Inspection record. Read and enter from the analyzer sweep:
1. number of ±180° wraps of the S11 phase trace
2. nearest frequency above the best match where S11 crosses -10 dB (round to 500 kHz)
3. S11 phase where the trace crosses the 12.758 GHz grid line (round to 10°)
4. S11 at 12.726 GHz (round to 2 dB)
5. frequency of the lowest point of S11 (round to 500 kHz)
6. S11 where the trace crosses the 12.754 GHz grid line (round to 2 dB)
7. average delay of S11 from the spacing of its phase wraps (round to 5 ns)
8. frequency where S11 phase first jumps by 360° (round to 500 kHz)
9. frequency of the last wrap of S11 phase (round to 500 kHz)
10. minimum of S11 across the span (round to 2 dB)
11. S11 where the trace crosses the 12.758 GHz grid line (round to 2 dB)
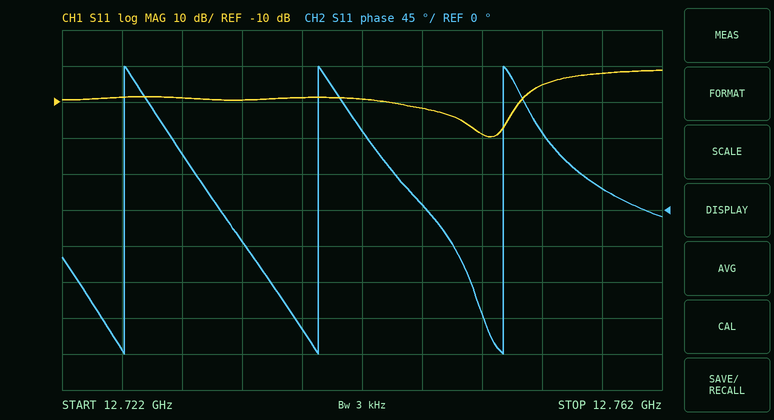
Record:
3
12.7525 GHz
30°
-8 dB
12.7505 GHz
-6 dB
80 ns
12.7260 GHz
12.7515 GHz
-20 dB
-2 dB
